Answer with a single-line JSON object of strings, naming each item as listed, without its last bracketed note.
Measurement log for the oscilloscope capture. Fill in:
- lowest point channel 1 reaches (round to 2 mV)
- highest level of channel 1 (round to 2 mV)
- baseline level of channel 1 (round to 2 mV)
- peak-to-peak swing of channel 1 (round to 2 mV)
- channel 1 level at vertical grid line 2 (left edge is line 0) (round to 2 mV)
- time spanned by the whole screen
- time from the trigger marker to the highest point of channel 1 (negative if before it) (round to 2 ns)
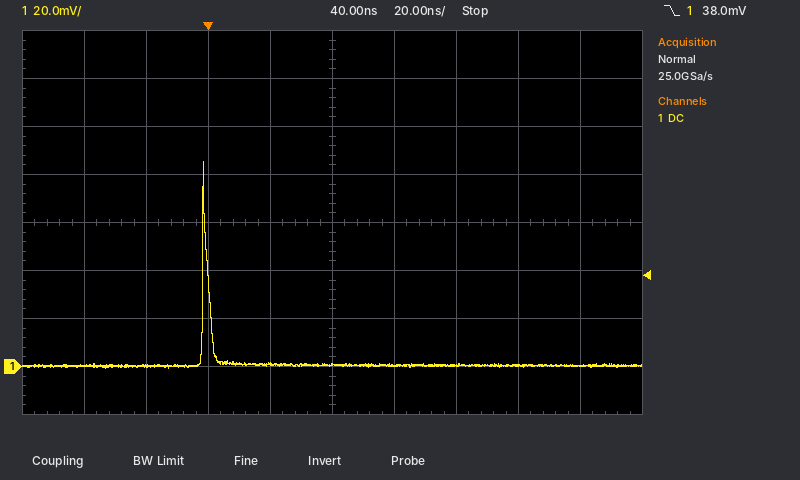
{"lowest point channel 1 reaches": "0 mV", "highest level of channel 1": "86 mV", "baseline level of channel 1": "0 mV", "peak-to-peak swing of channel 1": "86 mV", "channel 1 level at vertical grid line 2 (left edge is line 0)": "0 mV", "time spanned by the whole screen": "200 ns", "time from the trigger marker to the highest point of channel 1 (negative if before it)": "-2 ns"}
